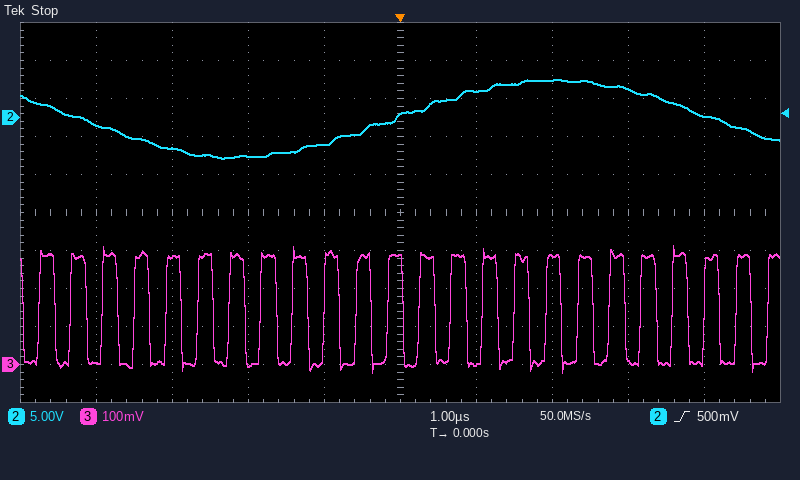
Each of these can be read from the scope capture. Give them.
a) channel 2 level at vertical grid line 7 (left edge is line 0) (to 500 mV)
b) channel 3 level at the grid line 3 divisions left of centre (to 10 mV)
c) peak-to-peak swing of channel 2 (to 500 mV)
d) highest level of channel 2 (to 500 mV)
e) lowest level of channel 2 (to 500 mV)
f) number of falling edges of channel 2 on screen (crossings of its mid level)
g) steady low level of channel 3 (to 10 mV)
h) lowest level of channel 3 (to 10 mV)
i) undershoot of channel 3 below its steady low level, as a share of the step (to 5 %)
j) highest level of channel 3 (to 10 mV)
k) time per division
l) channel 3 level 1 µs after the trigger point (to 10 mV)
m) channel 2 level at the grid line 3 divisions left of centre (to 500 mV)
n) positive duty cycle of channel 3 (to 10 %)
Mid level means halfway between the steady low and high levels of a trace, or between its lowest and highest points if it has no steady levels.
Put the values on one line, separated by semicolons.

5.0 V; 280 mV; 10.5 V; 5.0 V; -5.5 V; 2; 0 mV; -20 mV; 10 %; 310 mV; 1 µs; 0 mV; -4.0 V; 50 %
